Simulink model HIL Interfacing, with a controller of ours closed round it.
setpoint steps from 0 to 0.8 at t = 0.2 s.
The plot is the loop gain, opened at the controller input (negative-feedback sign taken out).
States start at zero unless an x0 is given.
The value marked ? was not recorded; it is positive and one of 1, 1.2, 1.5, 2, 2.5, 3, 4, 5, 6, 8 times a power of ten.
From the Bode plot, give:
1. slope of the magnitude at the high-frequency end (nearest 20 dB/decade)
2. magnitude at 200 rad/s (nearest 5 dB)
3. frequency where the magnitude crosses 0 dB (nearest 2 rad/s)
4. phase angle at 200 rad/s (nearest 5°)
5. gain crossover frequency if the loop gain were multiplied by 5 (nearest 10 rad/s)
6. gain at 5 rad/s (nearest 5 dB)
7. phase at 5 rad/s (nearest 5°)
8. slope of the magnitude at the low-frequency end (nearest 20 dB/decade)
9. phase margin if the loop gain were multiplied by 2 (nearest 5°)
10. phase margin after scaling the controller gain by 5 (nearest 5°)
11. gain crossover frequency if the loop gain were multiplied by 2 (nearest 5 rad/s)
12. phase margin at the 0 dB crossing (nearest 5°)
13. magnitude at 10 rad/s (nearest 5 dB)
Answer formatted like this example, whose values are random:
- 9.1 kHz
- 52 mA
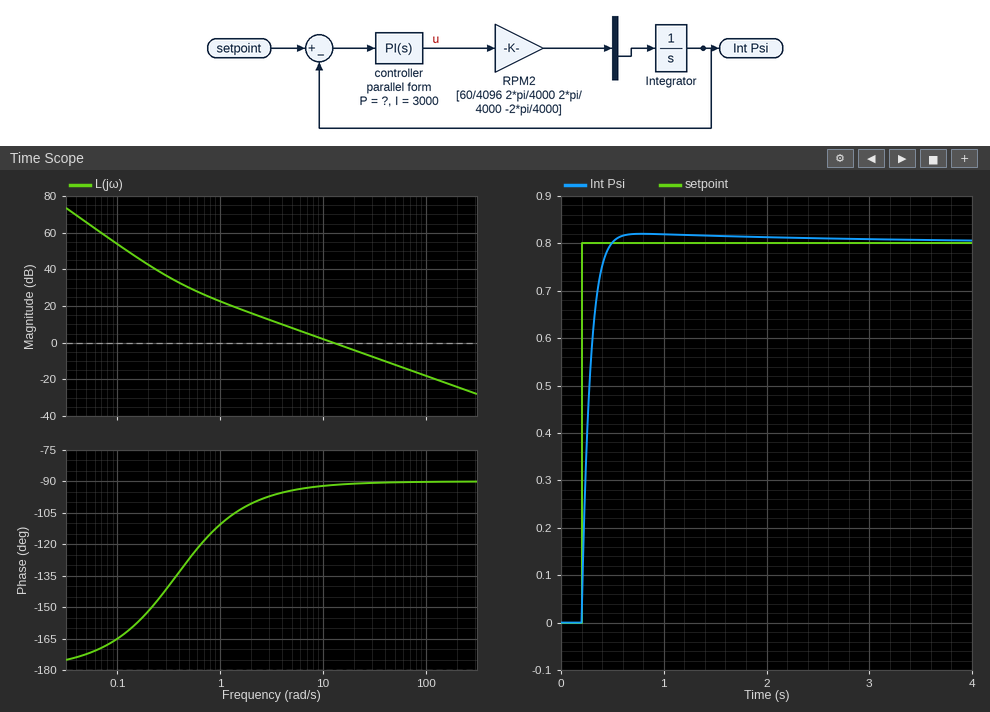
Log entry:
- -20 dB/decade
- -25 dB
- 12 rad/s
- -90°
- 60 rad/s
- 10 dB
- -95°
- -40 dB/decade
- 90°
- 90°
- 25 rad/s
- 90°
- 0 dB
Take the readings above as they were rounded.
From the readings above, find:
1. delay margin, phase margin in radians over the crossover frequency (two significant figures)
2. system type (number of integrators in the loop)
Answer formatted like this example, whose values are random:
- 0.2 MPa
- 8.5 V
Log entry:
- 0.13 s
- 2
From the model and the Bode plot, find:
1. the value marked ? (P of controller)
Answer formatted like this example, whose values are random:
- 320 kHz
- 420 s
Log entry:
- 8000
